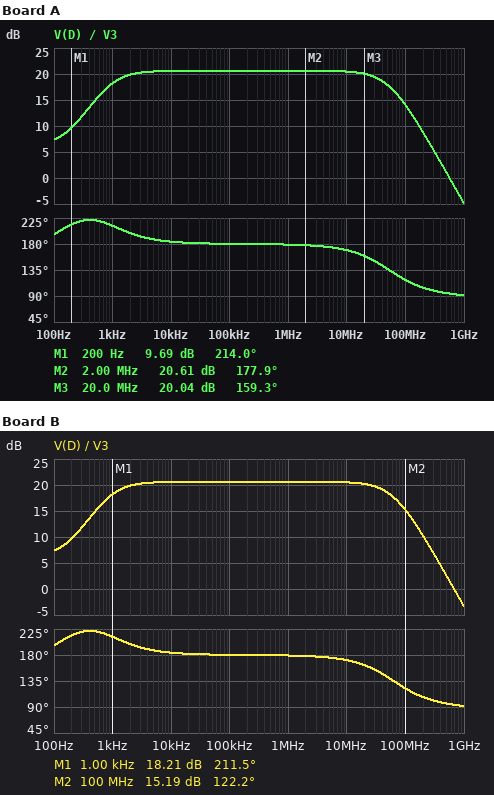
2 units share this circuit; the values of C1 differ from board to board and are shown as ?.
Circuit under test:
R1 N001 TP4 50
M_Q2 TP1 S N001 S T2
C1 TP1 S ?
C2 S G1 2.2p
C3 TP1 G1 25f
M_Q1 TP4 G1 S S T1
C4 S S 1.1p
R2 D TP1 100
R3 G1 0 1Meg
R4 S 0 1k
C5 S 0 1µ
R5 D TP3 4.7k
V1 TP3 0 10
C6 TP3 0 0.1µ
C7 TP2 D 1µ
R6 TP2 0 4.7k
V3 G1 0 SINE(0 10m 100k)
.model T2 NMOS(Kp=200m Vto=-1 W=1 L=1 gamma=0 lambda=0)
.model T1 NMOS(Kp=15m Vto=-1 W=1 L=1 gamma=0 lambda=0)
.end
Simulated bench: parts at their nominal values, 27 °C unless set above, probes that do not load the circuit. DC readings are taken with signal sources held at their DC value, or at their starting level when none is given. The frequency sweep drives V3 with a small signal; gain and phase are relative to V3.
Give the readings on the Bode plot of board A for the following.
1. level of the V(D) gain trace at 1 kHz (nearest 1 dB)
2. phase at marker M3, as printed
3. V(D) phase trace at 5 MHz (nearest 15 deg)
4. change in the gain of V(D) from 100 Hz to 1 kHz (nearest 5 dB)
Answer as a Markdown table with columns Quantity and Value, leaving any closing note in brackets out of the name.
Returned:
| Quantity | Value |
|---|---|
| level of the V(D) gain trace at 1 kHz | 18 dB |
| phase at marker M3, as printed | 159.3 deg |
| V(D) phase trace at 5 MHz | 180 deg |
| change in the gain of V(D) from 100 Hz to 1 kHz | 10 dB |
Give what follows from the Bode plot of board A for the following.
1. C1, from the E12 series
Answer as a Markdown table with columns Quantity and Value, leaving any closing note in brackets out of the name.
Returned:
| Quantity | Value |
|---|---|
| C1, from the E12 series | 1.2 pF |
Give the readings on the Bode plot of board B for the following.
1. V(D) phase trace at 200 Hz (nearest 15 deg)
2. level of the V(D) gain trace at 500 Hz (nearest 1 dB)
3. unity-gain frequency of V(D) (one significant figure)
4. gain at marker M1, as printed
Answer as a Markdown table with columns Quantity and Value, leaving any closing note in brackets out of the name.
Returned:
| Quantity | Value |
|---|---|
| V(D) phase trace at 200 Hz | 210 deg |
| level of the V(D) gain trace at 500 Hz | 15 dB |
| unity-gain frequency of V(D) | 700 MHz |
| gain at marker M1, as printed | 18.21 dB |
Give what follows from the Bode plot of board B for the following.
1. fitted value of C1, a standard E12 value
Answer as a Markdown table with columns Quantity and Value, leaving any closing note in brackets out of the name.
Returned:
| Quantity | Value |
|---|---|
| fitted value of C1, a standard E12 value | 1 pF |
